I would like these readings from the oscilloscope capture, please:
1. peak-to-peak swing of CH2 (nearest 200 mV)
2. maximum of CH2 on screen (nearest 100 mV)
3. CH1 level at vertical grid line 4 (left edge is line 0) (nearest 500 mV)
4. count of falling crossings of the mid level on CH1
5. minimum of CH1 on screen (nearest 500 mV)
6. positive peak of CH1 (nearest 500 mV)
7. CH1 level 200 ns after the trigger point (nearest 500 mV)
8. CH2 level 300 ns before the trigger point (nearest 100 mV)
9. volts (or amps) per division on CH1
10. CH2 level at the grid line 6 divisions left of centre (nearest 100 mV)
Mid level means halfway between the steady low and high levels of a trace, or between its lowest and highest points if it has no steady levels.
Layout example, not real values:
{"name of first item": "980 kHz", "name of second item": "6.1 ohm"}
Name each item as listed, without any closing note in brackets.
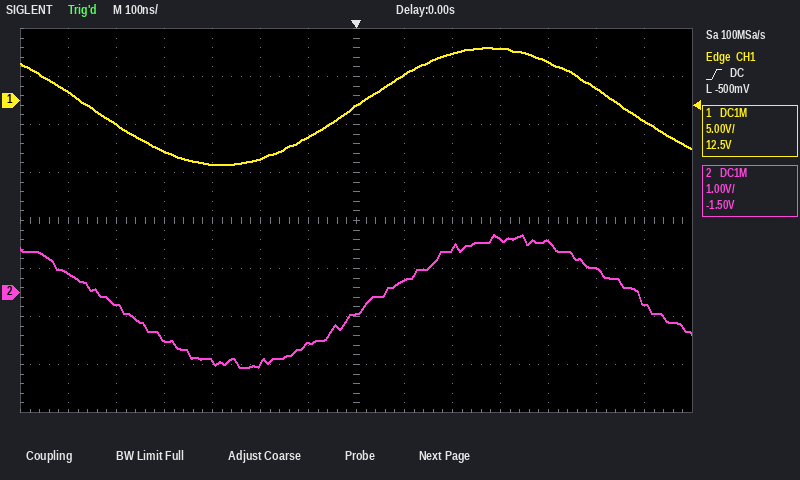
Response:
{"peak-to-peak swing of CH2": "2.8 V", "maximum of CH2 on screen": "1.2 V", "CH1 level at vertical grid line 4 (left edge is line 0)": "-6.5 V", "count of falling crossings of the mid level on CH1": "2", "minimum of CH1 on screen": "-6.5 V", "positive peak of CH1": "5.5 V", "CH1 level 200 ns after the trigger point": "5.0 V", "CH2 level 300 ns before the trigger point": "-1.4 V", "volts (or amps) per division on CH1": "5 V", "CH2 level at the grid line 6 divisions left of centre": "400 mV"}
